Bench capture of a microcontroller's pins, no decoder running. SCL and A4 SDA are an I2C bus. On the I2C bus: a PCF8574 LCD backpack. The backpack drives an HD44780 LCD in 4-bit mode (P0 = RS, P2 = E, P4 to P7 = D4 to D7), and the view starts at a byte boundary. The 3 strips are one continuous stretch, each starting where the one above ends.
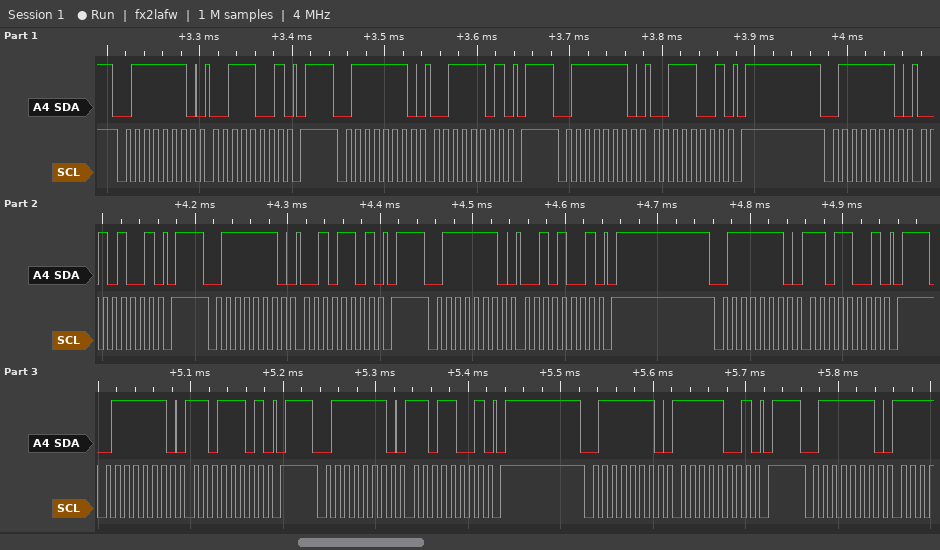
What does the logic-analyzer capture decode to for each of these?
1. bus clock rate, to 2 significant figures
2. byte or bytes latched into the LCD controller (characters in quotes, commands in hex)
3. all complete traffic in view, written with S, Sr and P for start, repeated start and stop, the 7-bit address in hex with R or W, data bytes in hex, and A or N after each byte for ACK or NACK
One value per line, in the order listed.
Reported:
100 kHz
'2'
S 3FW A 39 A P S 3FW A 3D A P S 3FW A 39 A P S 3FW A 29 A P S 3FW A 2D A P S 3FW A 29 A P S 3FW A D9 A P S 3FW A DD A P S 3FW A D9 A P S 3FW A F9 A P S 3FW A
